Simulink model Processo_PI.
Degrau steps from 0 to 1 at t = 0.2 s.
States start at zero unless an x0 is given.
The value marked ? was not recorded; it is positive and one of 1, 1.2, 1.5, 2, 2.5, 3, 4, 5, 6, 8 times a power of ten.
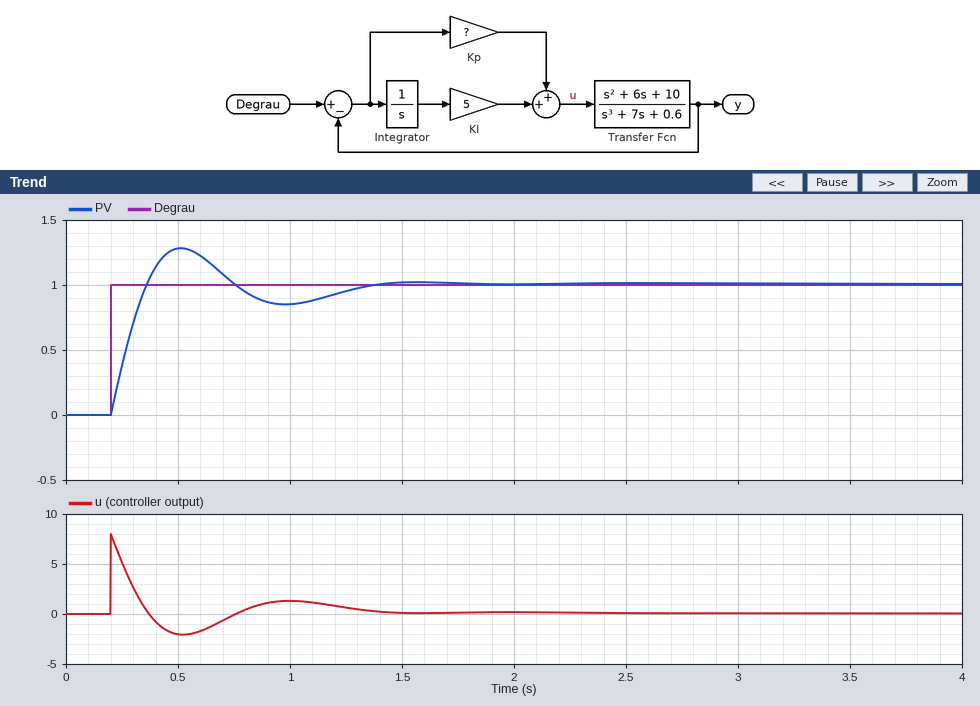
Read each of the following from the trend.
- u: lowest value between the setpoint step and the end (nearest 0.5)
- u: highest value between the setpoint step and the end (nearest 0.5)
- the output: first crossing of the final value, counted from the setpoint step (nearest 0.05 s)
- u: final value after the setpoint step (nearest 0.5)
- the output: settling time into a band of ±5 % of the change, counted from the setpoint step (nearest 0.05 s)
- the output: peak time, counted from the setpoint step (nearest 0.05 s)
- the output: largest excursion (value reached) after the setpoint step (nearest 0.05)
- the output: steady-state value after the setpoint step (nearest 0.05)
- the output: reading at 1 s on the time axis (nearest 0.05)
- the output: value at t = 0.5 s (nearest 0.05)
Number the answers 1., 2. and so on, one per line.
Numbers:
1. -2.0
2. 8.0
3. 0.15 s
4. 0.0
5. 1.05 s
6. 0.30 s
7. 1.30
8. 1.00
9. 0.85
10. 1.30
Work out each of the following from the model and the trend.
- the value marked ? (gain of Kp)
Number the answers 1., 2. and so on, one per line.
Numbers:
1. 8
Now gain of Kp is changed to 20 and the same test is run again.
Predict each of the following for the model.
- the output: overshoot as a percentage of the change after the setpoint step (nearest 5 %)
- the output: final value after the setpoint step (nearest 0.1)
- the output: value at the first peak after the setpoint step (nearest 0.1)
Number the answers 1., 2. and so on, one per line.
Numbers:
1. 15 %
2. 1.0
3. 1.2
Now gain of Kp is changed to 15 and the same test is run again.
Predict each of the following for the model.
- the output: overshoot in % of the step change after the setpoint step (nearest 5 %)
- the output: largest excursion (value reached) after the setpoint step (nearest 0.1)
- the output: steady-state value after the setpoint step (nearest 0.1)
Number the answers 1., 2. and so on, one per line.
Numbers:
1. 20 %
2. 1.2
3. 1.0
